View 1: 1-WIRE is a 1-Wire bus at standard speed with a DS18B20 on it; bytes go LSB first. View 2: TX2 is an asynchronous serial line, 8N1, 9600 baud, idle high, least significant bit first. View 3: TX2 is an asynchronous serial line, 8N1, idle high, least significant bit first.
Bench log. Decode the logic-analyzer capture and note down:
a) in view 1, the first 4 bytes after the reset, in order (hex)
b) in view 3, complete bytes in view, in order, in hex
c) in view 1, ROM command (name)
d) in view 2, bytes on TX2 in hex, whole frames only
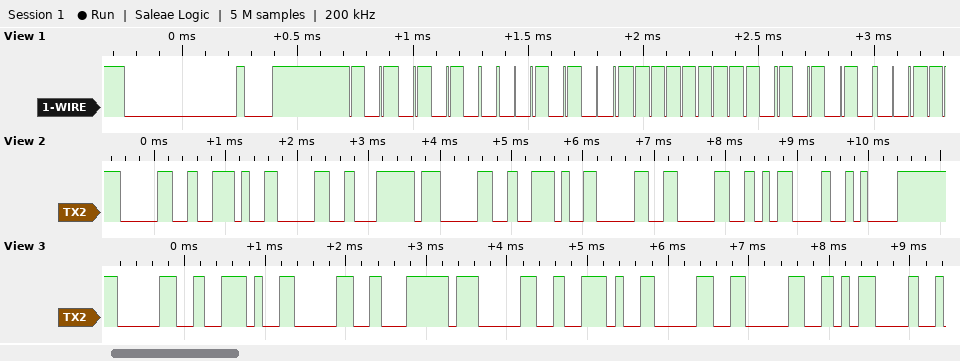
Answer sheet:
55 28 FF 55
0x30 0x2E 0x30 0x7C 0x30 0x2E 0x30 0x30 0x0D
Match ROM
30 2E 30 7C 30 2E 30 30 0D 0A
